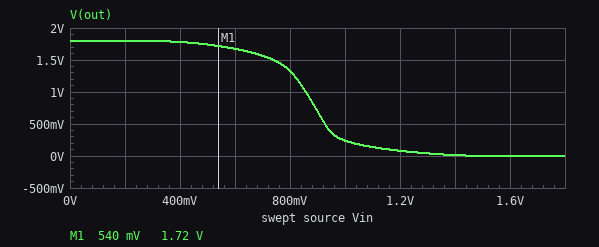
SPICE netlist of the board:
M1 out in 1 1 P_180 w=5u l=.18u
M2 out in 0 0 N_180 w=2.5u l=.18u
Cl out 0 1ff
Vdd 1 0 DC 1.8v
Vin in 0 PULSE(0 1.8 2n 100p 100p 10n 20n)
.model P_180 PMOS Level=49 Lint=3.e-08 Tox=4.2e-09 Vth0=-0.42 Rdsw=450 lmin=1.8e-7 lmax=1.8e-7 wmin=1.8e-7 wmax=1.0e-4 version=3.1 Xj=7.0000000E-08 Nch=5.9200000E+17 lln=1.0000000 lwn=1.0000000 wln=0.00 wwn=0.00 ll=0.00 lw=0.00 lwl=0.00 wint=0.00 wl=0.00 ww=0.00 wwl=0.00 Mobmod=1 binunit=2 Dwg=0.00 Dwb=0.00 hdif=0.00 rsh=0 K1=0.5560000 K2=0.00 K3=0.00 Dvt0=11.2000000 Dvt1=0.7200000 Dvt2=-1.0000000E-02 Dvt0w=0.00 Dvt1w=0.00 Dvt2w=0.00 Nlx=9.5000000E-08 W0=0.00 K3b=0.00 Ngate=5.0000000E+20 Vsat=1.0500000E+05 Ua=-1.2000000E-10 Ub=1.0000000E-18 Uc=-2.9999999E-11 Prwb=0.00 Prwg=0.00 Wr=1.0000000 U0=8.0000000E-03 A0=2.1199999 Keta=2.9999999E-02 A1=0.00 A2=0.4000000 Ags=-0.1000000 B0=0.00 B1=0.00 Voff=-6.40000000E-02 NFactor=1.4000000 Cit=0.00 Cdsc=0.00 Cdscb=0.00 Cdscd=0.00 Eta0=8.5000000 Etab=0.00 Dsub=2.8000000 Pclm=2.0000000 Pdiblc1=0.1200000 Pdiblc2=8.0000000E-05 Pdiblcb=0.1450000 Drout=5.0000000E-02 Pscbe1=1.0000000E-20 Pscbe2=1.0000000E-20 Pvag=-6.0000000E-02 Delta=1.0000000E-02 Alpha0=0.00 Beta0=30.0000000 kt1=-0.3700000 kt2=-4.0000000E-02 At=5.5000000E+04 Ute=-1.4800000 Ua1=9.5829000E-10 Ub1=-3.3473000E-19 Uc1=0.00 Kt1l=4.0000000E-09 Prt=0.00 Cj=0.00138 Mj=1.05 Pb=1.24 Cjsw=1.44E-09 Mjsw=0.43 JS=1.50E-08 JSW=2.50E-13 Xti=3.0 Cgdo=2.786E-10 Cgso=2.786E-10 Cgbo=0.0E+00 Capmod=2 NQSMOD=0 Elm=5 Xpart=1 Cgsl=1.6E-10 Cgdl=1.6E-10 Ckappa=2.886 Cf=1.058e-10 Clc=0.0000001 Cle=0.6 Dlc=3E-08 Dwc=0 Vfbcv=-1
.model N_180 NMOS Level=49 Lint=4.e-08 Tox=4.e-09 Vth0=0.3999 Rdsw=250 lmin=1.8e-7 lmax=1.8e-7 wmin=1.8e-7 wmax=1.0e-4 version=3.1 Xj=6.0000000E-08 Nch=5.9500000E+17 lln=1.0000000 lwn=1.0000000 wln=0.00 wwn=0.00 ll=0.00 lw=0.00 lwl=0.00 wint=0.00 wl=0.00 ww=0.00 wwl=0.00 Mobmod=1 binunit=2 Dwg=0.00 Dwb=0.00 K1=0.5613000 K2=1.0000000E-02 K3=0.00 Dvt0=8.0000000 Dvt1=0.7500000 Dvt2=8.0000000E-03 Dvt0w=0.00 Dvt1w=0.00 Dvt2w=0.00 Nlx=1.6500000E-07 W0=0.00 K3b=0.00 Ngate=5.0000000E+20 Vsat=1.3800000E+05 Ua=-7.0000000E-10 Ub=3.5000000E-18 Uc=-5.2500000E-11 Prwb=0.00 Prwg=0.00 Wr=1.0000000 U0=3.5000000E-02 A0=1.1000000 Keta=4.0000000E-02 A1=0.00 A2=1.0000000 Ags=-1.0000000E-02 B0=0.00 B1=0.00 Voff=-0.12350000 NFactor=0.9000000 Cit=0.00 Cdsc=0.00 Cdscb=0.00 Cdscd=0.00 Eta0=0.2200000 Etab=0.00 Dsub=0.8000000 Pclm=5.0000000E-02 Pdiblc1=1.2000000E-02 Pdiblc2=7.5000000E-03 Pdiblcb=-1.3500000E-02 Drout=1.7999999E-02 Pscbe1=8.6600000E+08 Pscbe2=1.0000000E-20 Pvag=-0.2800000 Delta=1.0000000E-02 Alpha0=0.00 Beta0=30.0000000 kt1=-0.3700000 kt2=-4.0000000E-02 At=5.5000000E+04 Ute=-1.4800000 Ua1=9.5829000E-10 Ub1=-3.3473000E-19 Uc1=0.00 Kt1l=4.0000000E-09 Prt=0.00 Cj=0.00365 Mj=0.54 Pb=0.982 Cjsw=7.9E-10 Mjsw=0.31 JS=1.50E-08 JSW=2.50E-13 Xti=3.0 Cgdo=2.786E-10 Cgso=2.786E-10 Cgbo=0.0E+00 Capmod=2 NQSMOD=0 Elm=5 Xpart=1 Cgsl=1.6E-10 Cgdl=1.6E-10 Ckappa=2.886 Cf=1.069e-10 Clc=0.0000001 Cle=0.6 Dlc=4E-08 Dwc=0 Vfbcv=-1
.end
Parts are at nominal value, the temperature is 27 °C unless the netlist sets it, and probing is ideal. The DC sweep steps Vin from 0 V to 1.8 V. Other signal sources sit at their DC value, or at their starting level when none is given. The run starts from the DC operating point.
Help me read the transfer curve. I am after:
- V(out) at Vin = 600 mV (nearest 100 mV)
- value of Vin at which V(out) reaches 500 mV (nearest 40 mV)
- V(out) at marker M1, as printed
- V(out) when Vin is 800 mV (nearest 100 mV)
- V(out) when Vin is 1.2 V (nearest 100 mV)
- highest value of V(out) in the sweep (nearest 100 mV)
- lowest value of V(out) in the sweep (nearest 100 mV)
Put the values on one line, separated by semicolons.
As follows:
1.7 V; 920 mV; 1.72 V; 1.3 V; 100 mV; 1.8 V; 0 V
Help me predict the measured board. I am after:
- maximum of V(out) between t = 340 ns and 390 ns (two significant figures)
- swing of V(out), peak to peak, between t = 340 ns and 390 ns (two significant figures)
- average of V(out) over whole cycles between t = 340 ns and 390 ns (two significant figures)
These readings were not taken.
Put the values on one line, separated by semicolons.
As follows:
1.8 V; 1.9 V; 890 mV
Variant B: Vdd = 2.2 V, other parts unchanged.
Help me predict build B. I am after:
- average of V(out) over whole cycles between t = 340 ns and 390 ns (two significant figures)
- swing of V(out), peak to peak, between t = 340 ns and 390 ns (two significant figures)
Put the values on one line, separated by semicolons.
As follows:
1.1 V; 2.2 V
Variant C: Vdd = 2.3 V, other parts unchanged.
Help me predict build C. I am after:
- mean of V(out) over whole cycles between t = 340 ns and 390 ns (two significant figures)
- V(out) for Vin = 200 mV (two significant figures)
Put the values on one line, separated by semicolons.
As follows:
1.2 V; 2.3 V
